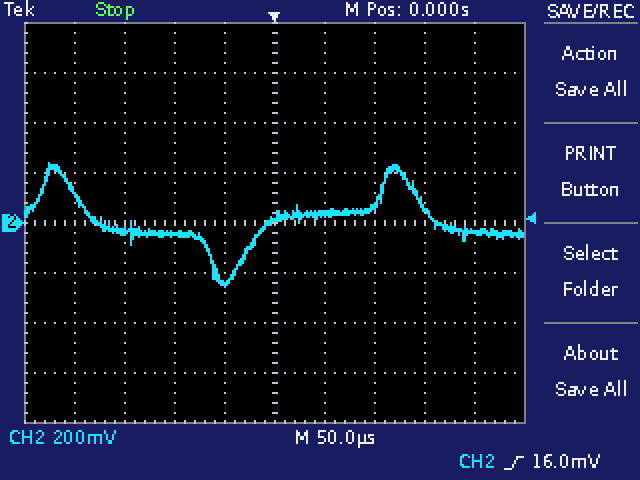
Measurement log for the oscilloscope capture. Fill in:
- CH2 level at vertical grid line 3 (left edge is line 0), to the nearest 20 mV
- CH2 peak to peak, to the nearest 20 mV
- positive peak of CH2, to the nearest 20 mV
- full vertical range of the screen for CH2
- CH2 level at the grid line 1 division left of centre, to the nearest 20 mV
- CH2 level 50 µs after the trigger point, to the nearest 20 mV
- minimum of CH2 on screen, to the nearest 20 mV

-40 mV
500 mV
240 mV
1.6 V
-240 mV
40 mV
-260 mV
